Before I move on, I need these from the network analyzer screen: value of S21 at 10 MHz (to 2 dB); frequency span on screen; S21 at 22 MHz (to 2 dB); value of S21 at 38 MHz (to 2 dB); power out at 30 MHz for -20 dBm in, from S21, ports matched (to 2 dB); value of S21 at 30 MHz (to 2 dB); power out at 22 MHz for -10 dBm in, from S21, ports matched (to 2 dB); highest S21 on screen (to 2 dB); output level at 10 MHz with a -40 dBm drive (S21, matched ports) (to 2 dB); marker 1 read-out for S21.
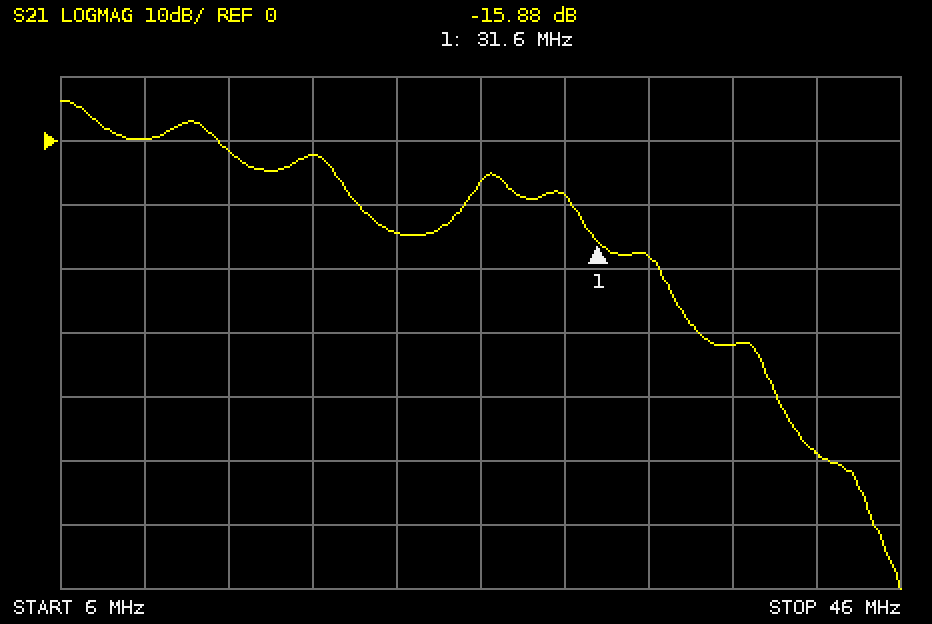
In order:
0 dB
40 MHz
-14 dB
-32 dB
-28 dBm
-8 dB
-24 dBm
6 dB
-40 dBm
-15.88 dB
